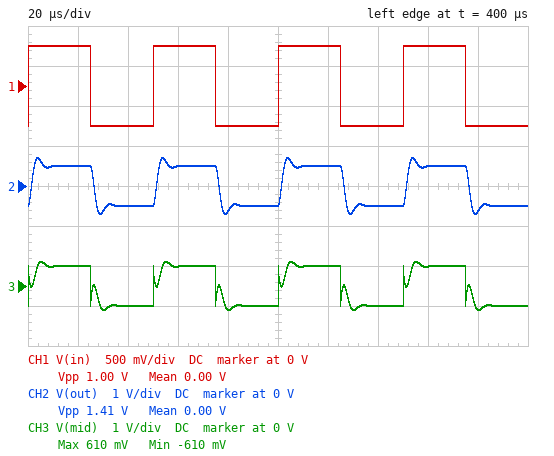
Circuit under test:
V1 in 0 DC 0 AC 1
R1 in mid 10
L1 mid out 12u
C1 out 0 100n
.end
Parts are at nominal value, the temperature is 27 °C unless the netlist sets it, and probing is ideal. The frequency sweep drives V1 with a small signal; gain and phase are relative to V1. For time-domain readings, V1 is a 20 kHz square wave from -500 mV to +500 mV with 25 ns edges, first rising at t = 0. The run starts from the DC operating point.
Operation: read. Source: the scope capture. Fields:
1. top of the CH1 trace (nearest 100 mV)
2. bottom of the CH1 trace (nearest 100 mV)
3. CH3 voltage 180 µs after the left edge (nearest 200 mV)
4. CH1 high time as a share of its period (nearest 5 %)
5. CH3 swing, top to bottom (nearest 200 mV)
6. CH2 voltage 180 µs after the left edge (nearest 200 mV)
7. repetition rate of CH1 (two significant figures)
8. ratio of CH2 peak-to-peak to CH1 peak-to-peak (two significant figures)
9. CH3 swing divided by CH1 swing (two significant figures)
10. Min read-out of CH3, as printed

500 mV
-500 mV
-600 mV
50 %
1.2 V
-600 mV
20 kHz
1.4
1.2
-610 mV
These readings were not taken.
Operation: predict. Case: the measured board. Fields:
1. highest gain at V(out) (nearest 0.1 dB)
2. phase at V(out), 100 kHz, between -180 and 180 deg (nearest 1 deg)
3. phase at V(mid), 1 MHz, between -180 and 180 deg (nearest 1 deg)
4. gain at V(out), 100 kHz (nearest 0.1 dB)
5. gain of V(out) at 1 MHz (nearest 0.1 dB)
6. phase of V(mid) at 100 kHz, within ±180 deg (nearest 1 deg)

1.8 dB
-50 deg
8 deg
1.7 dB
-33.4 dB
-50 deg
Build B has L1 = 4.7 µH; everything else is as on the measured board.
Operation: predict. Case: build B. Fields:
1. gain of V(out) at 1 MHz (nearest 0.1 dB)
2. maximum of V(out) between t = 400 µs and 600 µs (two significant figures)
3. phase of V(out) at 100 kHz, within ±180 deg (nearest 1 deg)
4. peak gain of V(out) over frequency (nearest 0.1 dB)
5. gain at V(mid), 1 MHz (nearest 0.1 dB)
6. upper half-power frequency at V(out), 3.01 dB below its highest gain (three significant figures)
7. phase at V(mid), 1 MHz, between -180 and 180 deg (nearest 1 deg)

-25.4 dB
540 mV
-38 deg
0 dB
-0.5 dB
225 kHz
20 deg
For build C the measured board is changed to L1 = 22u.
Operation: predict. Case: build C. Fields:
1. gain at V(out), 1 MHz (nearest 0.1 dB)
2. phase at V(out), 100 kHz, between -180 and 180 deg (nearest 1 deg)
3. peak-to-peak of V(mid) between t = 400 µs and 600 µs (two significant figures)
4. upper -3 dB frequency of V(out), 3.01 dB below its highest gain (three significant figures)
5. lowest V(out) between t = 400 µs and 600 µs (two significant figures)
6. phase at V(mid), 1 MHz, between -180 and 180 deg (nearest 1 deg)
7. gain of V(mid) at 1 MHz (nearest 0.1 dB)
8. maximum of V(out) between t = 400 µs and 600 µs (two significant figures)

-38.7 dB
-78 deg
1.3 V
127 kHz
-830 mV
4 deg
0 dB
830 mV
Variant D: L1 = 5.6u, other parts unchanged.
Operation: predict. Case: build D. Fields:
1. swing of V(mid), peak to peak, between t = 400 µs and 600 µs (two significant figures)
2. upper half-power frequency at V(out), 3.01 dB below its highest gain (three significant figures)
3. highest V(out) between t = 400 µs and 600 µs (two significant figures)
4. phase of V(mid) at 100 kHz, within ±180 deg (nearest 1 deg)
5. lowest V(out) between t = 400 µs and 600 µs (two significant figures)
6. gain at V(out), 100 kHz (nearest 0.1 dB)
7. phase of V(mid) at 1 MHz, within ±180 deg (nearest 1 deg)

1.1 V
223 kHz
560 mV
-39 deg
-560 mV
0 dB
17 deg
